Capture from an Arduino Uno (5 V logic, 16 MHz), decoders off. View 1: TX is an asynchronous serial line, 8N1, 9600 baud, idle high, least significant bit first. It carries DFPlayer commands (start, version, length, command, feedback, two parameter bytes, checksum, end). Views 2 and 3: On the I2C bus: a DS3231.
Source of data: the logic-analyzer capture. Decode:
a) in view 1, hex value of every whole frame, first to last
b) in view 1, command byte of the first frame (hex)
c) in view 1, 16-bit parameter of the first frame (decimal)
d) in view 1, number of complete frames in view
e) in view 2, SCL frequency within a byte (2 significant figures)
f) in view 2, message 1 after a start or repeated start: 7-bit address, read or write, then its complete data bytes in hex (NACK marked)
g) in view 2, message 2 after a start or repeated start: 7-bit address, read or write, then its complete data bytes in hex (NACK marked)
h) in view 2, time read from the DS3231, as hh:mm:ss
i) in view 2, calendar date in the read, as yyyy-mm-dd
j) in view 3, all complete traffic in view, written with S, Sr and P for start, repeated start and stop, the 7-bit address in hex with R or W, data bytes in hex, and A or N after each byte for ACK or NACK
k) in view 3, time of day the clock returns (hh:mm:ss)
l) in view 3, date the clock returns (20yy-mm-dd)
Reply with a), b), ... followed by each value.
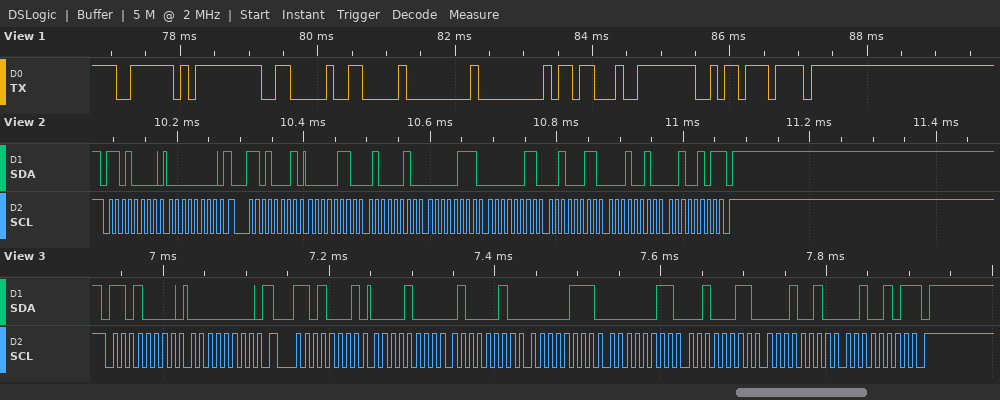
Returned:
a) 0x7E 0xFF 0x06 0x06 0x00 0x00 0x1B 0xFE 0xDA 0xEF
b) 0x06
c) 27
d) 10
e) 100 kHz
f) 0x68 write: 00
g) 0x68 read: 06 42 07 03 23 12 25 NACK
h) 07:42:06
i) 2025-12-23
j) S 68W A 00 A Sr 68R A 08 A 42 A 07 A 03 A 23 A 12 A 25 N P
k) 07:42:08
l) 2025-12-23
